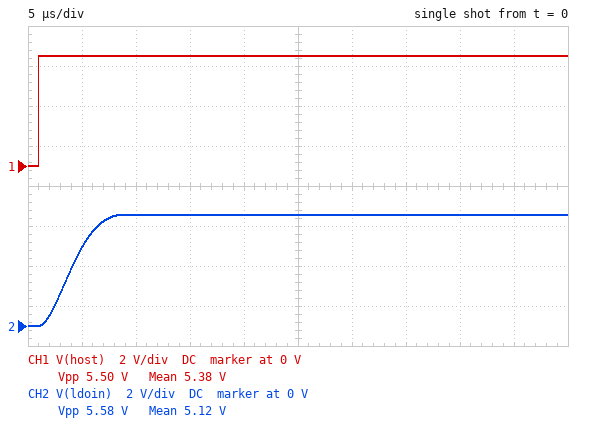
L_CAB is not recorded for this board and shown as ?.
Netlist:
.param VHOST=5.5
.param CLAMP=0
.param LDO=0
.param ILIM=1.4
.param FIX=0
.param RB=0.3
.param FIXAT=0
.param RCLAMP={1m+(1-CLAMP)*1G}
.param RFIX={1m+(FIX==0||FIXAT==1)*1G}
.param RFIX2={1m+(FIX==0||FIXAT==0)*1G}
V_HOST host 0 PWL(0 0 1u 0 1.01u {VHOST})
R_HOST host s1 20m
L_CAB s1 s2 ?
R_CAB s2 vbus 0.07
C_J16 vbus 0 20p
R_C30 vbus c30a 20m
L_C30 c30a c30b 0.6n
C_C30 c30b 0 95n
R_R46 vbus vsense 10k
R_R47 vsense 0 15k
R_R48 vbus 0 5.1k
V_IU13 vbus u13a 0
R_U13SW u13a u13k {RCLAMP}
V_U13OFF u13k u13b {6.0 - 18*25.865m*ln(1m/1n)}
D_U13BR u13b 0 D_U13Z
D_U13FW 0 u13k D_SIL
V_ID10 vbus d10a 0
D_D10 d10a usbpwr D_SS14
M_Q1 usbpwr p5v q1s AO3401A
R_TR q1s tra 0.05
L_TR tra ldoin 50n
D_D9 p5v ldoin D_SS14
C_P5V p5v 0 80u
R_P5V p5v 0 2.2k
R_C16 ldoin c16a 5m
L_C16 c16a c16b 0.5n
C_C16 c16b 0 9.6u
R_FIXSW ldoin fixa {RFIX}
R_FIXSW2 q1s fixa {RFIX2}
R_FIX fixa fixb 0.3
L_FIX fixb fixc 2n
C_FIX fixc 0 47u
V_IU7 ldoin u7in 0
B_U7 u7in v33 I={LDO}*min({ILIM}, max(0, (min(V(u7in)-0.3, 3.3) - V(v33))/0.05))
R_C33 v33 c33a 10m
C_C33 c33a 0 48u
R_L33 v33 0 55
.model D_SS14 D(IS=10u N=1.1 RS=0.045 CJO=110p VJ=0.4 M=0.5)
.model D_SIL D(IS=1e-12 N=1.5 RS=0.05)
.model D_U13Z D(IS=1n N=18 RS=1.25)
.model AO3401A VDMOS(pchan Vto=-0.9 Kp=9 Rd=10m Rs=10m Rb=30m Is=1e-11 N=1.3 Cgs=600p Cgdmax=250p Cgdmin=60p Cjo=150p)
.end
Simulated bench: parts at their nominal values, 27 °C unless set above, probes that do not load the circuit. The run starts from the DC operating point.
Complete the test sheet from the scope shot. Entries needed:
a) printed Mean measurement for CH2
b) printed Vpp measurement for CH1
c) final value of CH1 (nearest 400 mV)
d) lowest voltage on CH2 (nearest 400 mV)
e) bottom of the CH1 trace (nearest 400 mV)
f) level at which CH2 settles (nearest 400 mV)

5.12 V
5.50 V
5.6 V
0 V
0 V
5.6 V
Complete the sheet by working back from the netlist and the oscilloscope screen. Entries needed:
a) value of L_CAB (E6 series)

330 nH
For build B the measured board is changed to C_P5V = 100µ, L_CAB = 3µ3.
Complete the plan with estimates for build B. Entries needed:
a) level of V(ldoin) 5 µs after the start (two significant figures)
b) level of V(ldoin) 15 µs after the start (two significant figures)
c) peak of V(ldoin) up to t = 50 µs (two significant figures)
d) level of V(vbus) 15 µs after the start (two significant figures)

980 mV
6.6 V
7.7 V
7.5 V
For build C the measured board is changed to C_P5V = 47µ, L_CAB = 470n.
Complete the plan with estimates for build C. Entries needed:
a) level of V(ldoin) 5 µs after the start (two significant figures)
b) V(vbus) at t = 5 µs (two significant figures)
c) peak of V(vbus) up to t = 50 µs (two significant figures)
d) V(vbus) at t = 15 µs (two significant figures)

3.5 V
5.3 V
6.3 V
5.8 V
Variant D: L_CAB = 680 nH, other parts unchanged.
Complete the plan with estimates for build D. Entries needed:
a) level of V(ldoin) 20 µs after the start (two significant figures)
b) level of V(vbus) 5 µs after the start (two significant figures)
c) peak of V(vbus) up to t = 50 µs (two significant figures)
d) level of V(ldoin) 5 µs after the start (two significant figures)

6.2 V
4.9 V
6.6 V
3.0 V
